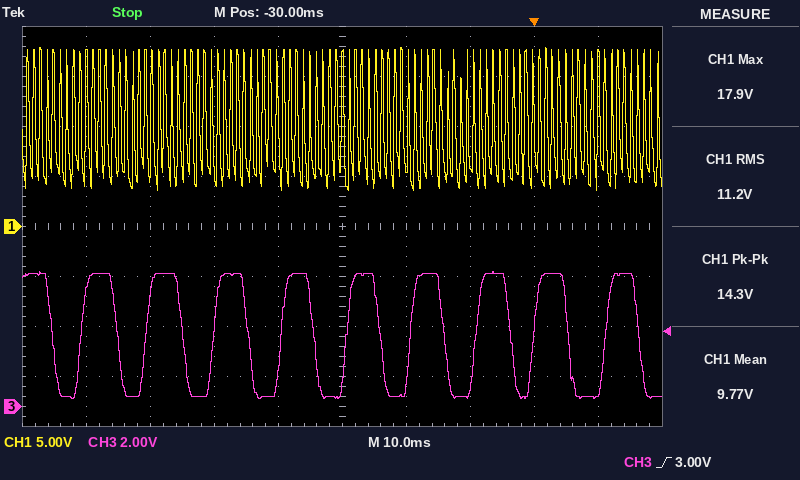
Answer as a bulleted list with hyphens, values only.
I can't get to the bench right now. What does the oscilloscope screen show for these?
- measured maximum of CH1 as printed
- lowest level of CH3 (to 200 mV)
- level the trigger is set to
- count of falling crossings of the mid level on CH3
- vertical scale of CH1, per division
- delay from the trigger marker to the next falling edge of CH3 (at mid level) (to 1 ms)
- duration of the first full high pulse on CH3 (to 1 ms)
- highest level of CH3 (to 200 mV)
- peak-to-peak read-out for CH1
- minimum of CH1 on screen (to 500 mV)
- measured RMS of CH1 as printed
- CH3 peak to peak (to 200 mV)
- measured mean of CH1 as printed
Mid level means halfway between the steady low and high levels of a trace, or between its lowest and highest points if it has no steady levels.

- 17.9 V
- 400 mV
- 3.00 V
- 10
- 5 V
- 5 ms
- 6 ms
- 5.4 V
- 14.3 V
- 3.5 V
- 11.2 V
- 5.0 V
- 9.77 V
